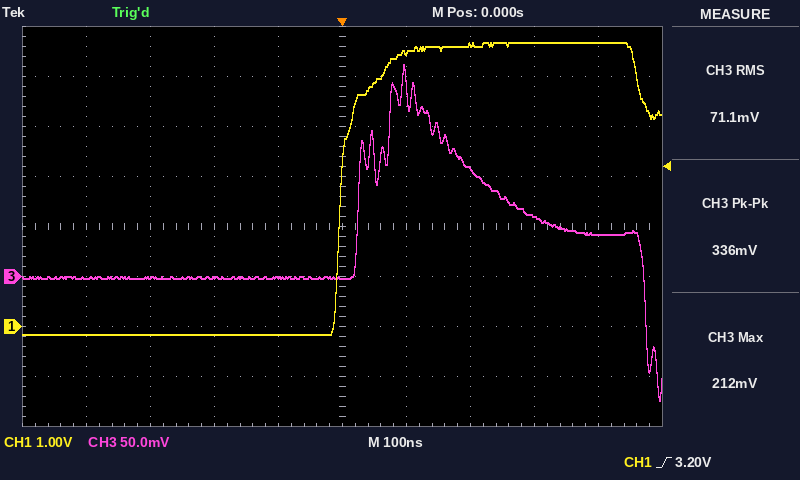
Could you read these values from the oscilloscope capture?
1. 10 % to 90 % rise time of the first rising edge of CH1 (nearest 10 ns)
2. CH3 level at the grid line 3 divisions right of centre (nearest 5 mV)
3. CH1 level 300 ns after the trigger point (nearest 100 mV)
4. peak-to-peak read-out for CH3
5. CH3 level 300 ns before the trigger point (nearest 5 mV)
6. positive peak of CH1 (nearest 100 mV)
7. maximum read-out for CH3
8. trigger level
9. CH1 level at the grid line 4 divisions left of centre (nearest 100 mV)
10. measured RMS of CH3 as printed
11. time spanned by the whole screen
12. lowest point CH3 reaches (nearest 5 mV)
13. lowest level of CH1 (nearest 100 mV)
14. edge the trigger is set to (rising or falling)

80 ns
60 mV
5.7 V
336 mV
0 mV
5.7 V
212 mV
3.20 V
-200 mV
71.1 mV
1 µs
-125 mV
-200 mV
rising
